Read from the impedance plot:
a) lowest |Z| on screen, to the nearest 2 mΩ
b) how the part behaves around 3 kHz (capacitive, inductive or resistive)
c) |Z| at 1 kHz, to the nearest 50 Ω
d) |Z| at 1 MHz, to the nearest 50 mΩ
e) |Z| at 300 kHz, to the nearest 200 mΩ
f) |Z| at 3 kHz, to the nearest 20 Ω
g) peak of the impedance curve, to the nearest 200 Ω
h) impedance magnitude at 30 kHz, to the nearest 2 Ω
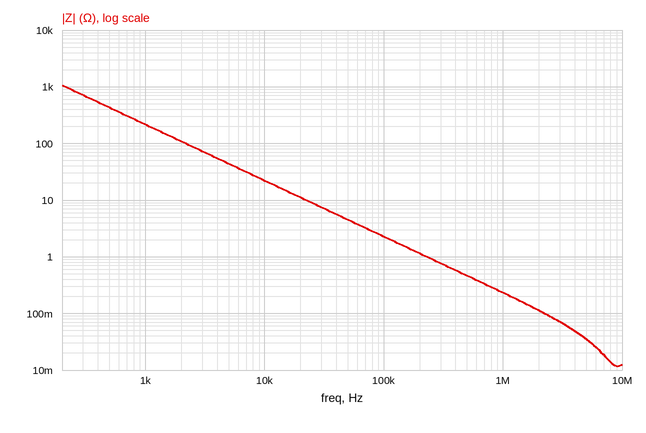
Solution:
12 mΩ
capacitive
200 Ω
250 mΩ
800 mΩ
80 Ω
1.0 kΩ
8 Ω
